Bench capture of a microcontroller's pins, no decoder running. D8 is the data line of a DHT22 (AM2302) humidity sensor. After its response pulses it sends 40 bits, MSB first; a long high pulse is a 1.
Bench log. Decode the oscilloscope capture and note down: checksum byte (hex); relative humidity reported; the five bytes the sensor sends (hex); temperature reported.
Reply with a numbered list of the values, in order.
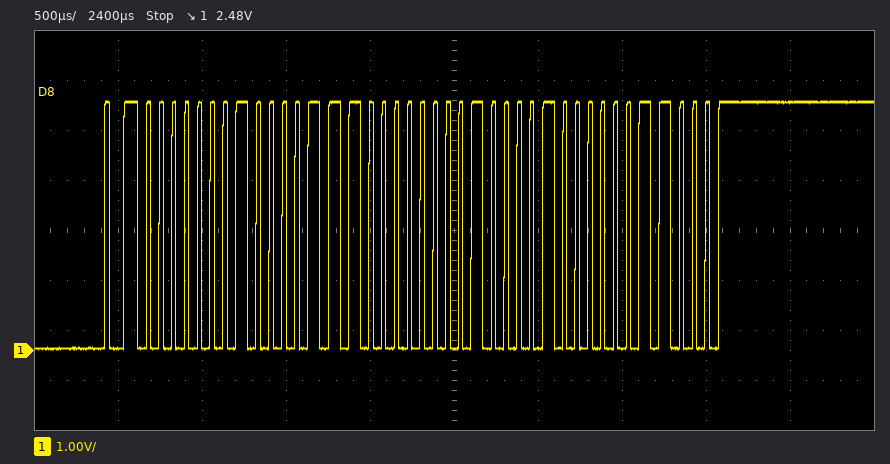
1. 0x18
2. 27.0 %
3. 01 0E 01 08 18
4. 26.4 °C
